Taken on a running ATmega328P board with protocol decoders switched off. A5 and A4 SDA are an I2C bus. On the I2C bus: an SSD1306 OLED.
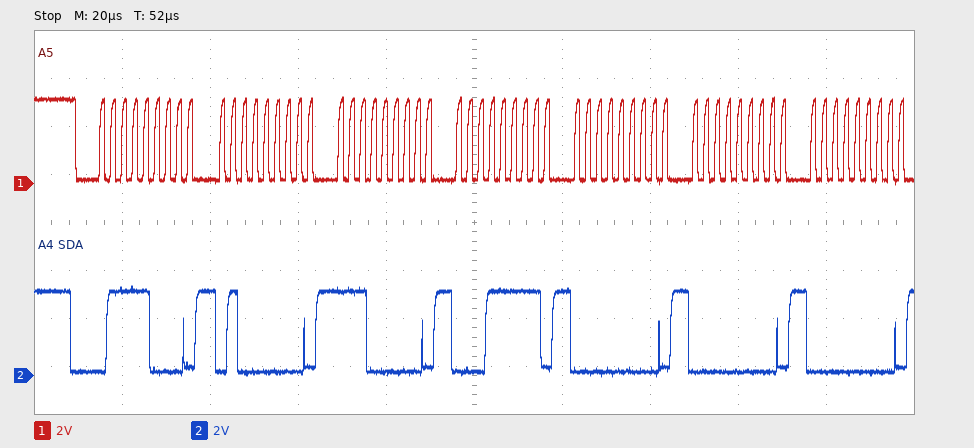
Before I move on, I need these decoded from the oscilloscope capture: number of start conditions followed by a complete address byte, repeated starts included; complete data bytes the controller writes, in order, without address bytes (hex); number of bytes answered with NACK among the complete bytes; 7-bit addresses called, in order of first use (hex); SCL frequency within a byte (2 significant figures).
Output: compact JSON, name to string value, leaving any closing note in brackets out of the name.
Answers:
{"number of start conditions followed by a complete address byte, repeated starts included": "1", "complete data bytes the controller writes, in order, without address bytes": "40 E0 1F 00 00 00", "number of bytes answered with NACK among the complete bytes": "0", "7-bit addresses called, in order of first use": "0x3C", "SCL frequency within a byte": "400 kHz"}
